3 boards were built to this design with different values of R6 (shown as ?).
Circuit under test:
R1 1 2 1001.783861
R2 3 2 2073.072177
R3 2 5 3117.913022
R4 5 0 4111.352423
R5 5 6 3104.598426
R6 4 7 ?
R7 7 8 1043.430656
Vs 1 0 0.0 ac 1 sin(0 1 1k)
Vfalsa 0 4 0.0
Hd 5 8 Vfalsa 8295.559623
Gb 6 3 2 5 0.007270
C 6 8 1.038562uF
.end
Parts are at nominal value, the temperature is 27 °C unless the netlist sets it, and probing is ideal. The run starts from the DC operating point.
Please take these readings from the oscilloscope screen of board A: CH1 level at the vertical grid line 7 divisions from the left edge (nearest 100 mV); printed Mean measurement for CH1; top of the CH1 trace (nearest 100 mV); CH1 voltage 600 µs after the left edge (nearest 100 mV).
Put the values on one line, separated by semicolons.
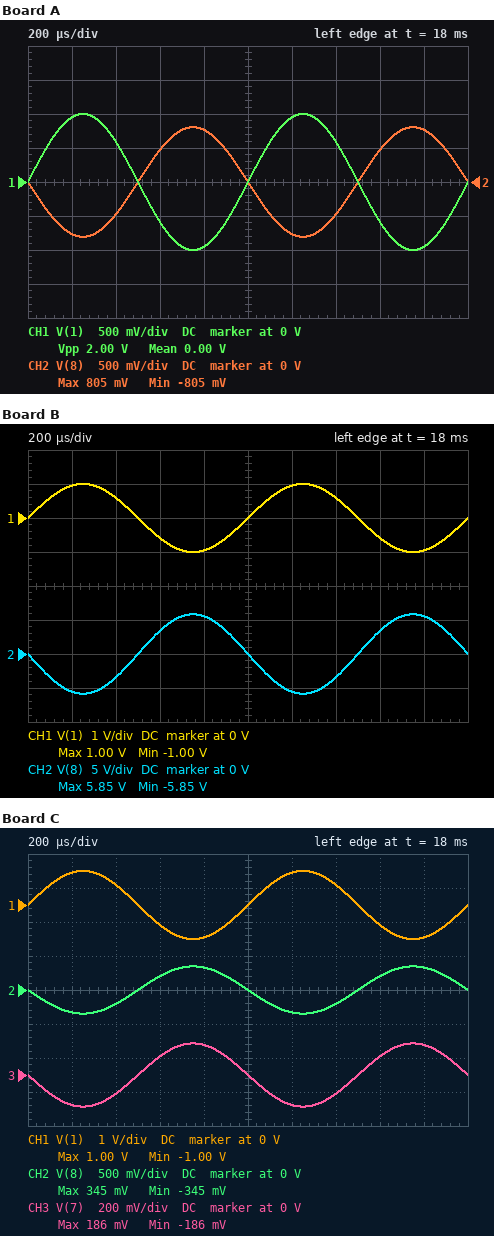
600 mV; 0.00 V; 1.0 V; -600 mV
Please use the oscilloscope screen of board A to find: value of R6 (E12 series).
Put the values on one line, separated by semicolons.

2.7 kΩ
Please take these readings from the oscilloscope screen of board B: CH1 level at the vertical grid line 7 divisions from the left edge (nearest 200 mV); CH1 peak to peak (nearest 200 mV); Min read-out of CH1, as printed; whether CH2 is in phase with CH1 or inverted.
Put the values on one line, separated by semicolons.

600 mV; 2.0 V; -1.00 V; inverted
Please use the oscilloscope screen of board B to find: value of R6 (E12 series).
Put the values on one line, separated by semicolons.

5.6 kΩ
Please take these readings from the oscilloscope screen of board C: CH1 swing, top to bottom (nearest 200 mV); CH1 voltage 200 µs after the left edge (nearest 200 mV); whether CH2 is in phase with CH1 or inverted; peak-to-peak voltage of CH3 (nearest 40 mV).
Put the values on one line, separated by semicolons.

2.0 V; 1.0 V; inverted; 360 mV
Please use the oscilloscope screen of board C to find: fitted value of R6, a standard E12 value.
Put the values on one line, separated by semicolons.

1.2 kΩ
